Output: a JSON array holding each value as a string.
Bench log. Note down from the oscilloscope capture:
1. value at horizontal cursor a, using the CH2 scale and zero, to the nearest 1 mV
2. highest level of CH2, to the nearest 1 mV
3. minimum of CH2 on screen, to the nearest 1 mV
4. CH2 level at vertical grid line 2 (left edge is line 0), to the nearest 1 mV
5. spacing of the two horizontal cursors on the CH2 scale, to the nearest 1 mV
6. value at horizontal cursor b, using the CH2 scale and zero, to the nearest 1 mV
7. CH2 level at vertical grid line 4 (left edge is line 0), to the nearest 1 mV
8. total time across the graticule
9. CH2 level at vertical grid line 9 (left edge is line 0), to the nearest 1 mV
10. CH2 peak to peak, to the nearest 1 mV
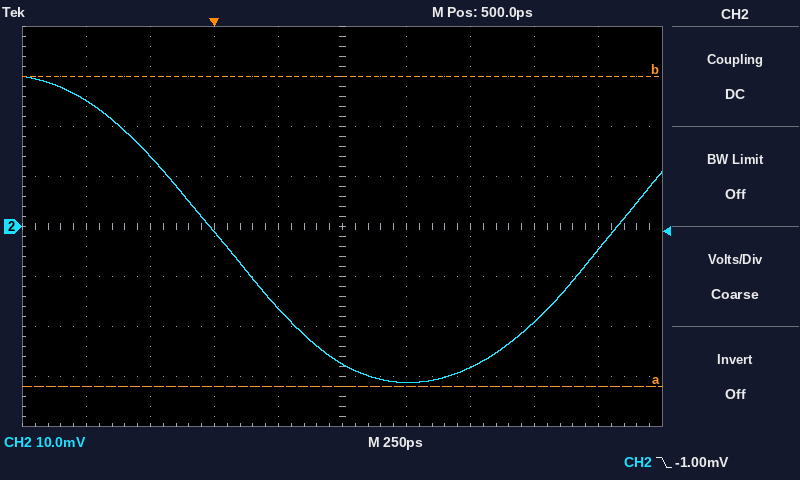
["-32 mV", "30 mV", "-31 mV", "14 mV", "62 mV", "30 mV", "-16 mV", "2.5 ns", "-5 mV", "61 mV"]
